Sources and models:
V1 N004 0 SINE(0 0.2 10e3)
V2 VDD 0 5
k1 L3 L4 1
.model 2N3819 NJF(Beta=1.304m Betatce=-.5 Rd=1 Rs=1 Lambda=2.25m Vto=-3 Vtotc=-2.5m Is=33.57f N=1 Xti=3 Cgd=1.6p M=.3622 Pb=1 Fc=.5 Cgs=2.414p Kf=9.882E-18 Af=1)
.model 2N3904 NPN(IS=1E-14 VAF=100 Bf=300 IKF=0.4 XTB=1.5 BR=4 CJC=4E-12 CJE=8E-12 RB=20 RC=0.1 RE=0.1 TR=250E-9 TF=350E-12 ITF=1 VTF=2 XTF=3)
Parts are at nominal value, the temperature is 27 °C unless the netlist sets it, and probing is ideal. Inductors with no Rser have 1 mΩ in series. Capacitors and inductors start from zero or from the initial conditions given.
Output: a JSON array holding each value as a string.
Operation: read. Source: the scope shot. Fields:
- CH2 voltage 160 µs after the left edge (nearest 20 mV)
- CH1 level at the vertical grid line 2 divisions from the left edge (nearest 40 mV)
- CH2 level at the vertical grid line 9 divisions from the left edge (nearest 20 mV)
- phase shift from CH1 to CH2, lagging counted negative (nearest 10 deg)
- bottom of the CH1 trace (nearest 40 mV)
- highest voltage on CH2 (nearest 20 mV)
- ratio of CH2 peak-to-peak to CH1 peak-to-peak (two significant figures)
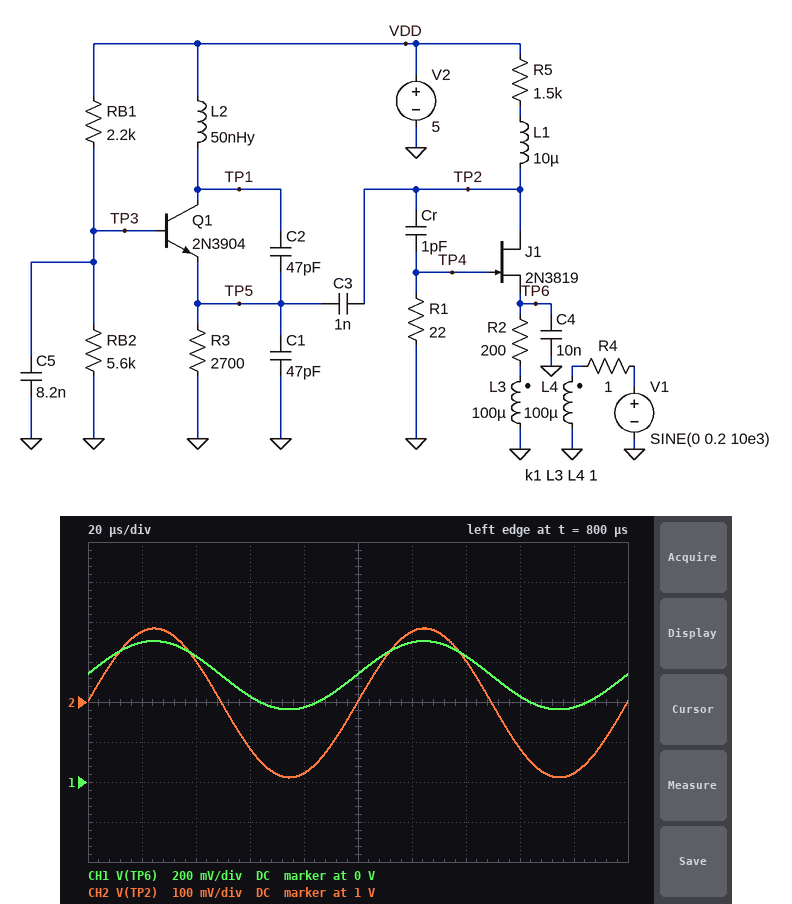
["880 mV", "640 mV", "820 mV", "0 deg", "360 mV", "1.18 V", "1.1"]
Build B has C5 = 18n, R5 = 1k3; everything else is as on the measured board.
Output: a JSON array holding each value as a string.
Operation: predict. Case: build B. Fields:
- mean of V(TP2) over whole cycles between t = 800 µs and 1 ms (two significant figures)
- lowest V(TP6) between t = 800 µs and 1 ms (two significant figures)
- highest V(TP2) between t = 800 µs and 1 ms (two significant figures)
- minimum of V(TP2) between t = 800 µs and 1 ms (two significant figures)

["1.1 V", "430 mV", "1.3 V", "950 mV"]
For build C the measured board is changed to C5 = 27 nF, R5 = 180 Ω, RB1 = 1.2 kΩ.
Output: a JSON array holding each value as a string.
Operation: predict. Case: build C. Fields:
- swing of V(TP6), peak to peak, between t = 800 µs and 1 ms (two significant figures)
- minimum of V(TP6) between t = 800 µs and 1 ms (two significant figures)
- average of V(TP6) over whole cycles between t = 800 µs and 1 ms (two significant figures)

["190 mV", "930 mV", "1.0 V"]
